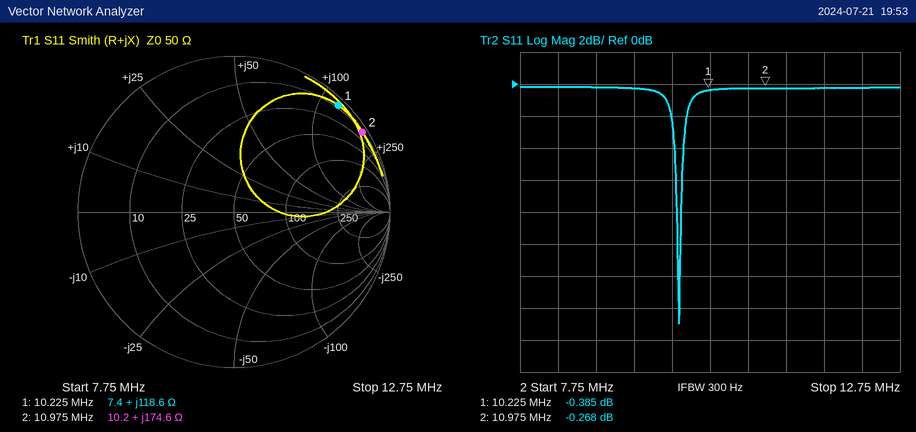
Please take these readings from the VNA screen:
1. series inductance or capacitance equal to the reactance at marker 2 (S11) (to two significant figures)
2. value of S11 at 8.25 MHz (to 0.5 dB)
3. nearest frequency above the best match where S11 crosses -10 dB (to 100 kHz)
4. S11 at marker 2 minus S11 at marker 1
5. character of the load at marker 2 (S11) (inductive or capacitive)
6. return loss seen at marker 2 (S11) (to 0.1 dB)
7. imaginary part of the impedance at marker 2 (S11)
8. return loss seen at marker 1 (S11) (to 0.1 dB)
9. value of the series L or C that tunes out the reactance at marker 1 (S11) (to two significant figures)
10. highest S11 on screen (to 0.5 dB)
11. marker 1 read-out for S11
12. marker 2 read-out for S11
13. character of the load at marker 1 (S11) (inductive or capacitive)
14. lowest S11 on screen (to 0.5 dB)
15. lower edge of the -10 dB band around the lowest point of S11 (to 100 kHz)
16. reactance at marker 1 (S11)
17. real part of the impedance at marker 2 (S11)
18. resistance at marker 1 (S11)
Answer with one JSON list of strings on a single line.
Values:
["2.5 µH", "0.0 dB", "9.9 MHz", "0.117 dB", "inductive", "0.3 dB", "+174.6 Ω", "0.4 dB", "130 pF", "0.0 dB", "-0.385 dB", "-0.268 dB", "inductive", "-15.0 dB", "9.8 MHz", "+118.6 Ω", "10.2 Ω", "7.4 Ω"]
